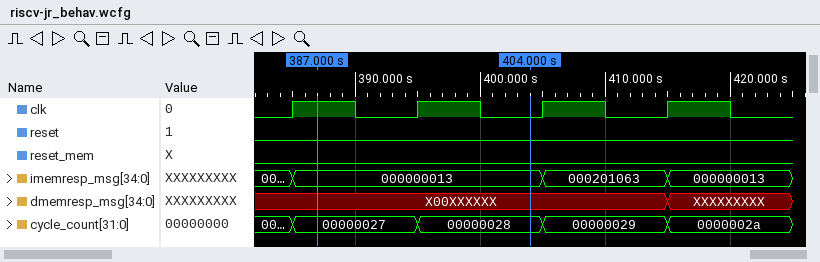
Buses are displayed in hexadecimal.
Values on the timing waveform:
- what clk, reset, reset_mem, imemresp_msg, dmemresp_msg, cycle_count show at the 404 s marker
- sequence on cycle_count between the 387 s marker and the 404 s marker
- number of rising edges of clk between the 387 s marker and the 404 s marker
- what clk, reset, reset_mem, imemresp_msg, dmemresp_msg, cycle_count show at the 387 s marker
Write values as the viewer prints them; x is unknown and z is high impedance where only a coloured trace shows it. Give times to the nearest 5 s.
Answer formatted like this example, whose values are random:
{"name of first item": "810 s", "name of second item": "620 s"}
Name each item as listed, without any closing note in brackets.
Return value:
{"what clk, reset, reset_mem, imemresp_msg, dmemresp_msg, cycle_count show at the 404 s marker": "clk=0, reset=0, reset_mem=0, imemresp_msg=000000013, dmemresp_msg=X00XXXXXX, cycle_count=00000028", "sequence on cycle_count between the 387 s marker and the 404 s marker": "00000027, 00000028", "number of rising edges of clk between the 387 s marker and the 404 s marker": "1", "what clk, reset, reset_mem, imemresp_msg, dmemresp_msg, cycle_count show at the 387 s marker": "clk=1, reset=0, reset_mem=0, imemresp_msg=000000013, dmemresp_msg=X00XXXXXX, cycle_count=00000027"}
